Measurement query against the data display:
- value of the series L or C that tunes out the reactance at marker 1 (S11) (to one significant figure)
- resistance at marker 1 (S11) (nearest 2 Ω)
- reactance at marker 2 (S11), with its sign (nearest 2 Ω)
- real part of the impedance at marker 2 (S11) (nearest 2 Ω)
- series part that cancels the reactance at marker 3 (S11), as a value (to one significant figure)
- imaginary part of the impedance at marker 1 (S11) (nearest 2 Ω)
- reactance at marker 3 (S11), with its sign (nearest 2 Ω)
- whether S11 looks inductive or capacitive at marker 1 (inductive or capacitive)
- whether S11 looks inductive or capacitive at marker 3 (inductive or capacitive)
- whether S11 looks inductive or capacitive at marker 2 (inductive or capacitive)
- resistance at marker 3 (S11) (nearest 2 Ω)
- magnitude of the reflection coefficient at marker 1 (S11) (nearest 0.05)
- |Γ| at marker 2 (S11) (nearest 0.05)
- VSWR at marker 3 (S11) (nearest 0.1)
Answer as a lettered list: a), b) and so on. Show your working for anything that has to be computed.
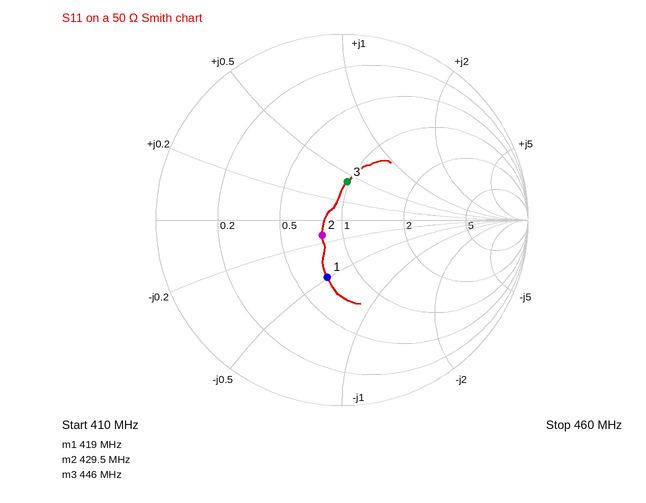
a) L = 24 Ω/(2π × 419 MHz) ≈ 9 nH
b) 36 Ω
c) -6 Ω
d) 40 Ω
e) C = 1/(2π × 446 MHz × 20 Ω) ≈ 17.8 pF, so 20 pF to one significant figure
f) -24 Ω
g) +20 Ω
h) capacitive
i) inductive
j) capacitive
k) 48 Ω
l) 0.30
m) 0.15
n) 1.5
